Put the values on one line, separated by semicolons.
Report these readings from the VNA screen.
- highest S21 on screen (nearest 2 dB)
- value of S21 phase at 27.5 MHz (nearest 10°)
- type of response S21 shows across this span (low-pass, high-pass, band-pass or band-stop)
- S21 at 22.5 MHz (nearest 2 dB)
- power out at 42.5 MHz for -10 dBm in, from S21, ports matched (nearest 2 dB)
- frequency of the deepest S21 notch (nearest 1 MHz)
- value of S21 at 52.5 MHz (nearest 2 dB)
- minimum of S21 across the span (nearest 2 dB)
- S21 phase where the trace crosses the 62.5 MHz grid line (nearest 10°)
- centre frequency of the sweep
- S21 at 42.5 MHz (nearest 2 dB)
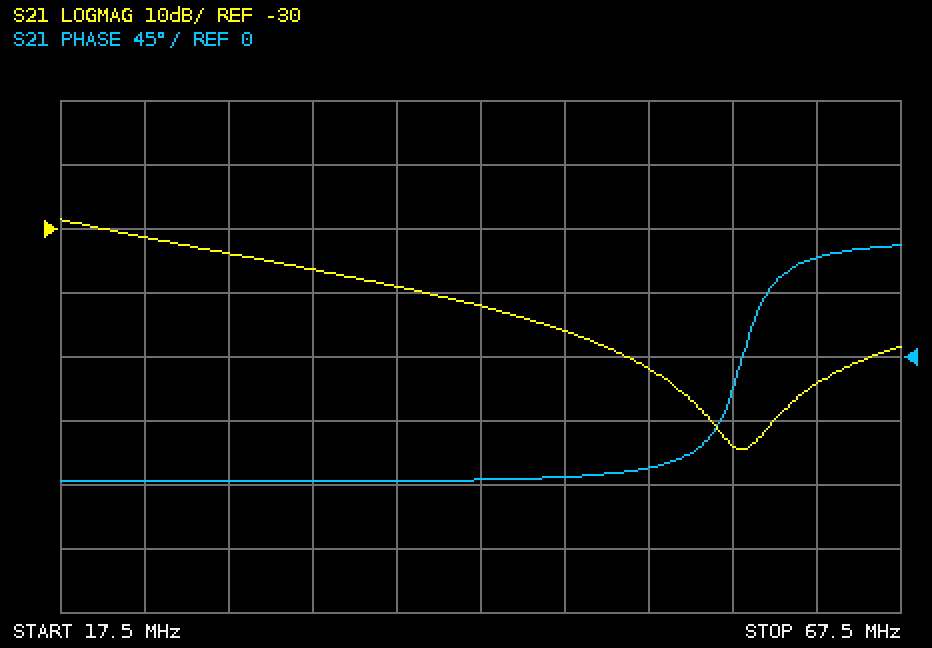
-28 dB; -90°; low-pass; -32 dB; -52 dBm; 58 MHz; -52 dB; -64 dB; 70°; 42.5 MHz; -42 dB
